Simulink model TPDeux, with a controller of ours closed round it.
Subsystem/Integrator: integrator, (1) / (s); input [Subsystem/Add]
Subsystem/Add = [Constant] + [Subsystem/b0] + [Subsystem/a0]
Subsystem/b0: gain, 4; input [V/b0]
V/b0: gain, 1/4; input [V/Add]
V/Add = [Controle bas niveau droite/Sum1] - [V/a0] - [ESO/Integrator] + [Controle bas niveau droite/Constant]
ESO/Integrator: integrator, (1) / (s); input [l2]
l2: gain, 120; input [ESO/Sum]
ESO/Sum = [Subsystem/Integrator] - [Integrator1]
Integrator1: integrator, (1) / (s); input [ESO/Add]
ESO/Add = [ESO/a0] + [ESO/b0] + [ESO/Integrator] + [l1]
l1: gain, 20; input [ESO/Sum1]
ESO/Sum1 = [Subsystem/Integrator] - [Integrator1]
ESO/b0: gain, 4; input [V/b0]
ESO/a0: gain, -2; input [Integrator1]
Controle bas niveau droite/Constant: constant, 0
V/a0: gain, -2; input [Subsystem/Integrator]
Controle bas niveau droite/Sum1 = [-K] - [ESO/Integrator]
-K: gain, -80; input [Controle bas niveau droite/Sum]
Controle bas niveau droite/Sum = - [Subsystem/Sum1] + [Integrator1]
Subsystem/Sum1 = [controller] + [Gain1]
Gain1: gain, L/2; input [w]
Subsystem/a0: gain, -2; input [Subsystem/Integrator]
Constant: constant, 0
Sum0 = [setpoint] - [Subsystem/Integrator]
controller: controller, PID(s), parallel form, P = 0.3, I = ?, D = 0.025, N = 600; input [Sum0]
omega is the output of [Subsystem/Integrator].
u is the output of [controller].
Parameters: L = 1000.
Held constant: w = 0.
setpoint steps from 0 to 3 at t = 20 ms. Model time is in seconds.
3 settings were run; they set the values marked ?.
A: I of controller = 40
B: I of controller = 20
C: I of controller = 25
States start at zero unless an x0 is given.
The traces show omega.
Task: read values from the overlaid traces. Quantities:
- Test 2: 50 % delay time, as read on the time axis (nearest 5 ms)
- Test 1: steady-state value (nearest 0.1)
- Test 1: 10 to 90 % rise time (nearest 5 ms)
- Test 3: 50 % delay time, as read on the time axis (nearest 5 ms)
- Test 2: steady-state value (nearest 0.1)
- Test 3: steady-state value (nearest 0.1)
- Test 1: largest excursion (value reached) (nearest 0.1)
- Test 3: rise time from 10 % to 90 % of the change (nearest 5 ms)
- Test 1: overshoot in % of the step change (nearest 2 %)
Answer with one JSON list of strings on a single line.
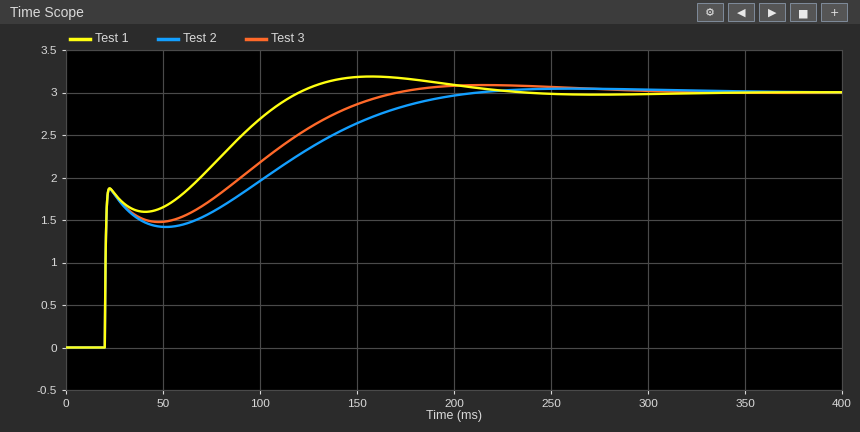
["20 ms", "3.0", "80 ms", "20 ms", "3.0", "3.0", "3.2", "115 ms", "6 %"]
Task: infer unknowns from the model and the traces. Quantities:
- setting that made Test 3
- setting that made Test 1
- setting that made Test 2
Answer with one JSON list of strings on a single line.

["C", "A", "B"]
